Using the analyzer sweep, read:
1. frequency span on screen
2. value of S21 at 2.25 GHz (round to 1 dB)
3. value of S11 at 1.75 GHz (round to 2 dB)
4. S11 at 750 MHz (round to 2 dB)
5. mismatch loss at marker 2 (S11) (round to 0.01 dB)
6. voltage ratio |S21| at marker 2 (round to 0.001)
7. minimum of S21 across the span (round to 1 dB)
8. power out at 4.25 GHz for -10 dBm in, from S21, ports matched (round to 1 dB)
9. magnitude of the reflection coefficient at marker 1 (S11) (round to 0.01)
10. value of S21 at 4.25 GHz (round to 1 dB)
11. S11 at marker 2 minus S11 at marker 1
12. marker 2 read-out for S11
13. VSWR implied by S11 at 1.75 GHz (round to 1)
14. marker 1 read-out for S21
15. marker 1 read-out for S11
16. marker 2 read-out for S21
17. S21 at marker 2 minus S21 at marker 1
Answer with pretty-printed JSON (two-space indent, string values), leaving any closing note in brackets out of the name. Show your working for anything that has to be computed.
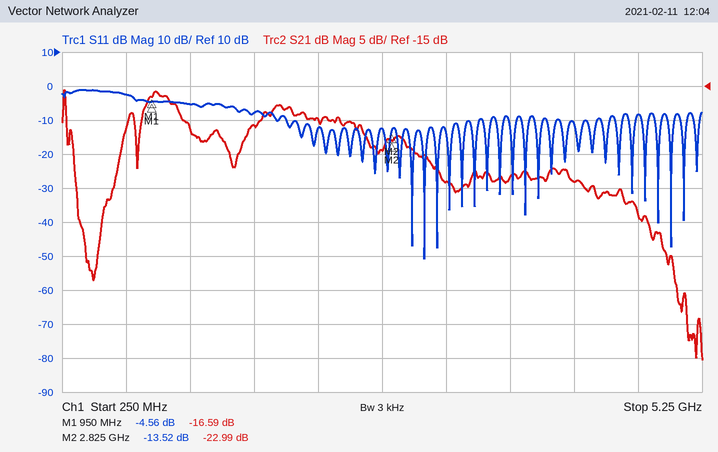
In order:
{
  "frequency span on screen": "5 GHz",
  "value of S21 at 2.25 GHz": "-20 dB",
  "value of S11 at 1.75 GHz": "-8 dB",
  "S11 at 750 MHz": "-2 dB",
  "mismatch loss at marker 2 (S11)": "−10 log10(1 − 10^(-13.52/10)) ≈ 0.20 dB",
  "voltage ratio |S21| at marker 2": "10^(-22.99/20) ≈ 0.071",
  "minimum of S21 across the span": "-55 dB",
  "power out at 4.25 GHz for -10 dBm in, from S21, ports matched": "-10 dBm + (-29 dB) = -39 dBm",
  "magnitude of the reflection coefficient at marker 1 (S11)": "10^(-4.56/20) ≈ 0.59",
  "value of S21 at 4.25 GHz": "-29 dB",
  "S11 at marker 2 minus S11 at marker 1": "-13.52 − (-4.56) = -8.96 dB",
  "marker 2 read-out for S11": "-13.52 dB",
  "VSWR implied by S11 at 1.75 GHz": "|Γ| = 10^(-8/20) = 0.3981; VSWR = (1 + 0.3981)/(1 − 0.3981) ≈ 2",
  "marker 1 read-out for S21": "-16.59 dB",
  "marker 1 read-out for S11": "-4.56 dB",
  "marker 2 read-out for S21": "-22.99 dB",
  "S21 at marker 2 minus S21 at marker 1": "-22.99 − (-16.59) = -6.40 dB"
}
